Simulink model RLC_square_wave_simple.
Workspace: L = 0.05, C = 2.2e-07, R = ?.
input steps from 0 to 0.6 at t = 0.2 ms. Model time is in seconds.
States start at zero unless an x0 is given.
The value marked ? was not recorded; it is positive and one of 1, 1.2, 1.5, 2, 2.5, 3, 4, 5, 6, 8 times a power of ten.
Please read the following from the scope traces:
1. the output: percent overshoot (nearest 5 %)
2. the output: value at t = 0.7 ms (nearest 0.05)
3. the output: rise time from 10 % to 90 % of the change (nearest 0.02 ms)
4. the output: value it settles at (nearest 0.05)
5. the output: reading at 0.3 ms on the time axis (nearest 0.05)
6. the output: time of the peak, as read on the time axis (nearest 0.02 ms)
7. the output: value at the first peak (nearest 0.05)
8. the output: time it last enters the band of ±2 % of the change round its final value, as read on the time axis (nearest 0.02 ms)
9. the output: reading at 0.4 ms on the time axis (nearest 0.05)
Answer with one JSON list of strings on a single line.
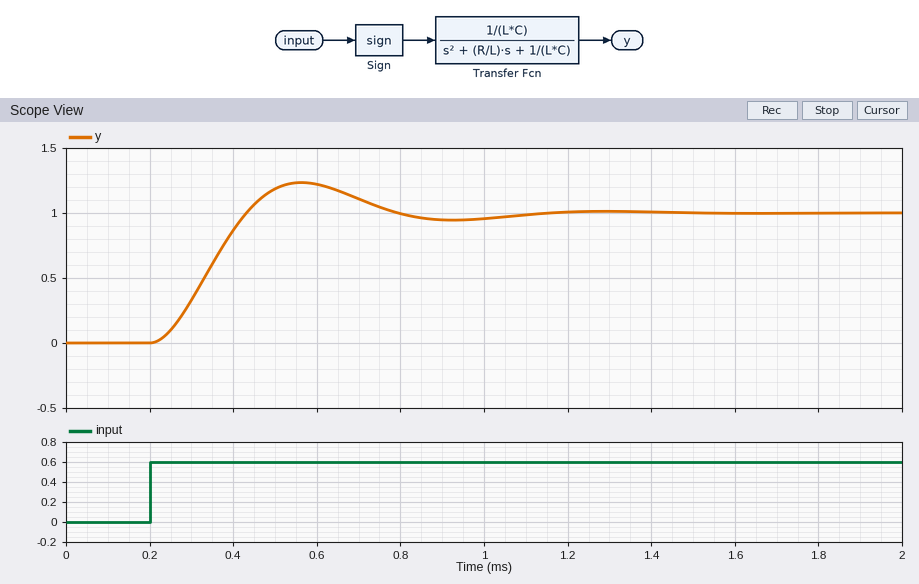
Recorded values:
["25 %", "1.10", "0.16 ms", "1.00", "0.35", "0.56 ms", "1.25", "1.08 ms", "0.85"]
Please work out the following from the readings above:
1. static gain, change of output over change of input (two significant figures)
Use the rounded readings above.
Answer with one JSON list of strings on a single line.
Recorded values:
["1.7"]
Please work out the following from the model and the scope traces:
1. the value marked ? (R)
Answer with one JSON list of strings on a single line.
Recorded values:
["400"]
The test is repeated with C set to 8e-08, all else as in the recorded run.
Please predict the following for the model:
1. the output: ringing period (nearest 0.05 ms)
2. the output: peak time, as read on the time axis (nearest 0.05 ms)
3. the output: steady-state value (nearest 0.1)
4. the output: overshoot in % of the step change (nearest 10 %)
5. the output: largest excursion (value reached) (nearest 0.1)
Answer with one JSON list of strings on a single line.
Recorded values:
["0.40 ms", "0.40 ms", "1.0", "40 %", "1.4"]
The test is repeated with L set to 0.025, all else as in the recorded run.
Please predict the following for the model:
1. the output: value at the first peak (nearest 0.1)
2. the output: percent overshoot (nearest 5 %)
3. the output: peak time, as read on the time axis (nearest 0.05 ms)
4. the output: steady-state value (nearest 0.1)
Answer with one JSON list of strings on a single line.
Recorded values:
["1.1", "10 %", "0.50 ms", "1.0"]
